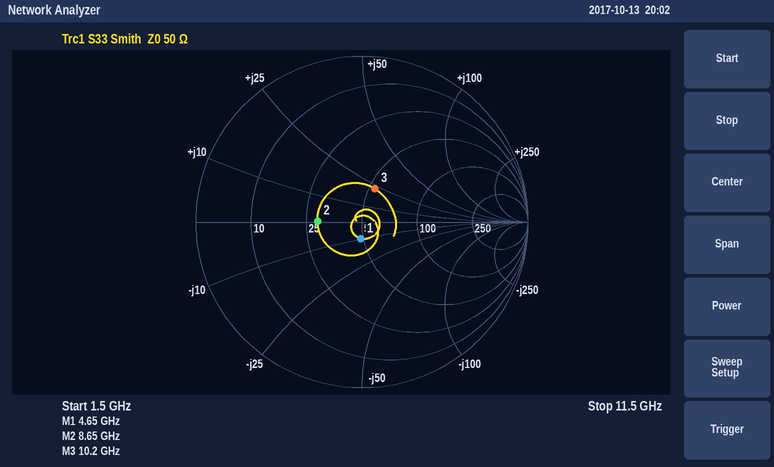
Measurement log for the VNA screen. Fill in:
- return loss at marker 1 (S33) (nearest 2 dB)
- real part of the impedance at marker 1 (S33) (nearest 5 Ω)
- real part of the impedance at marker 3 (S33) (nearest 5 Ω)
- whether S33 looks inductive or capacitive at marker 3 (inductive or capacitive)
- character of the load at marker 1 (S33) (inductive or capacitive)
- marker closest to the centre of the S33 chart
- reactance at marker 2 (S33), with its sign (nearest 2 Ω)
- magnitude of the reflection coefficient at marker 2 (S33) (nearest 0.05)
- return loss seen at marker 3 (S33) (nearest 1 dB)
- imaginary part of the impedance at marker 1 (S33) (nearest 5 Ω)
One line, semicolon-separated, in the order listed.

20 dB; 50 Ω; 55 Ω; inductive; capacitive; marker 1; 0 Ω; 0.25; 13 dB; -10 Ω
